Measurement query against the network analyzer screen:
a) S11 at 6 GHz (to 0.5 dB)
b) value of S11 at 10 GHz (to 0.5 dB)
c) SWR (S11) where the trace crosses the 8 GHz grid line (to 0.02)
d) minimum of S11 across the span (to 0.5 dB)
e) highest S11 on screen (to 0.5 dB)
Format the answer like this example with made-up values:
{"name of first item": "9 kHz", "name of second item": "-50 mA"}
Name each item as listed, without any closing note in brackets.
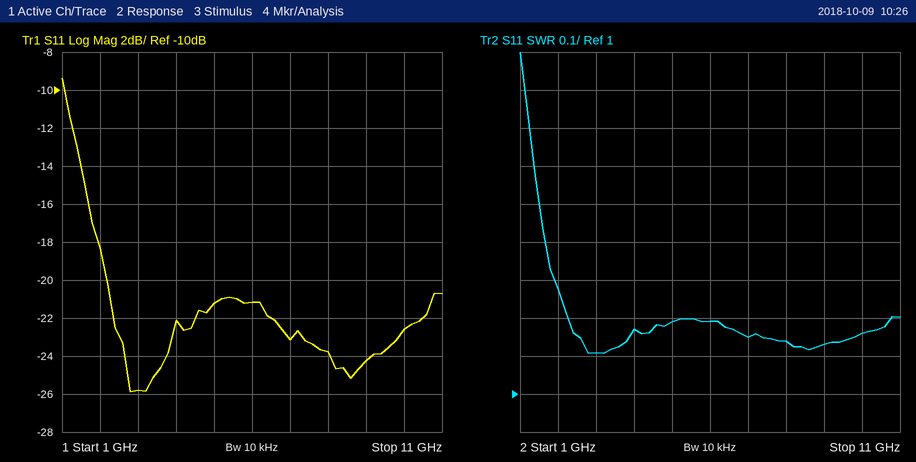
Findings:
{"S11 at 6 GHz": "-21.0 dB", "value of S11 at 10 GHz": "-22.5 dB", "SWR (S11) where the trace crosses the 8 GHz grid line": "1.14", "minimum of S11 across the span": "-26.0 dB", "highest S11 on screen": "-9.5 dB"}
